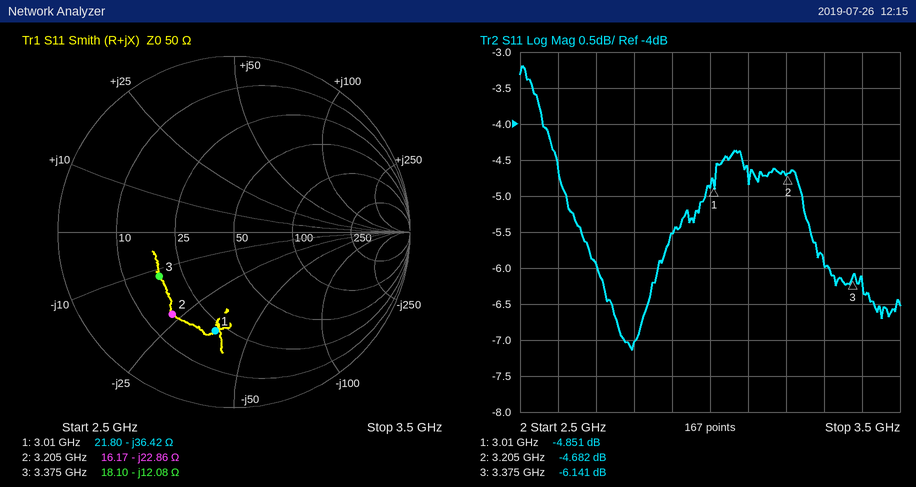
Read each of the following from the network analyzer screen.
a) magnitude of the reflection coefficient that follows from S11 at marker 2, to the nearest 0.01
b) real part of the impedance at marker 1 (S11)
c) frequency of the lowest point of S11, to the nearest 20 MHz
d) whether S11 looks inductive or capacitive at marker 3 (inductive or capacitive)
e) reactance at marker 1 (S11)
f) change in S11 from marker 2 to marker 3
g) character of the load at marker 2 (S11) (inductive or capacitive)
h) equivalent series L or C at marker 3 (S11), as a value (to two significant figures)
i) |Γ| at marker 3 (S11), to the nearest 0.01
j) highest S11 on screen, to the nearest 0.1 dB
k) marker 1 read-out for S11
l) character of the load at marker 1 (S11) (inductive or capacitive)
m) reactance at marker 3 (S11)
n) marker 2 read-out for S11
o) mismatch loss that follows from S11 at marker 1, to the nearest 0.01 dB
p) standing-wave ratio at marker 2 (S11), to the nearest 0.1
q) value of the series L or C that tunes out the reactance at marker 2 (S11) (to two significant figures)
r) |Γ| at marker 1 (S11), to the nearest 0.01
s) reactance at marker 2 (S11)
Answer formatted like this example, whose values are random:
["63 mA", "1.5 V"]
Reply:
["0.58", "21.80 Ω", "2.80 GHz", "capacitive", "-36.42 Ω", "-1.459 dB", "capacitive", "3.9 pF", "0.49", "-3.2 dB", "-4.851 dB", "capacitive", "-12.08 Ω", "-4.682 dB", "1.72 dB", "3.8", "1.1 nH", "0.57", "-22.86 Ω"]
